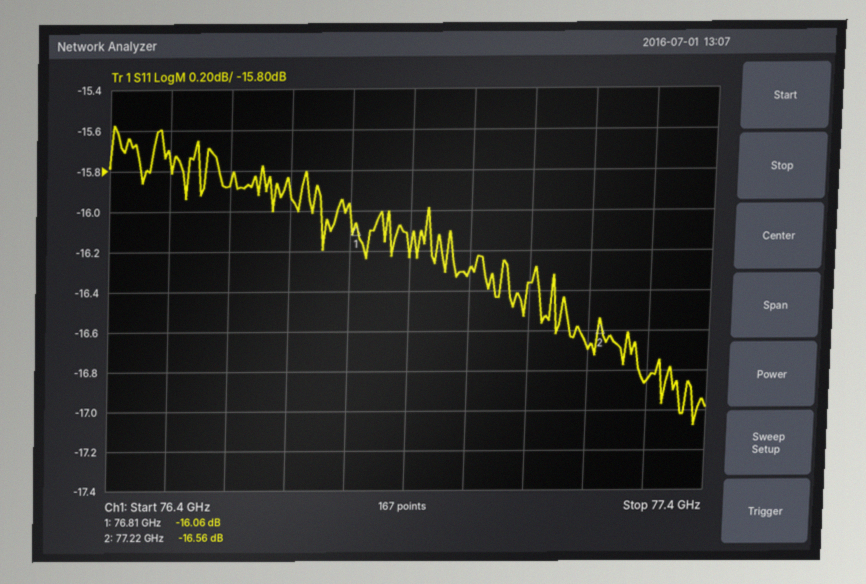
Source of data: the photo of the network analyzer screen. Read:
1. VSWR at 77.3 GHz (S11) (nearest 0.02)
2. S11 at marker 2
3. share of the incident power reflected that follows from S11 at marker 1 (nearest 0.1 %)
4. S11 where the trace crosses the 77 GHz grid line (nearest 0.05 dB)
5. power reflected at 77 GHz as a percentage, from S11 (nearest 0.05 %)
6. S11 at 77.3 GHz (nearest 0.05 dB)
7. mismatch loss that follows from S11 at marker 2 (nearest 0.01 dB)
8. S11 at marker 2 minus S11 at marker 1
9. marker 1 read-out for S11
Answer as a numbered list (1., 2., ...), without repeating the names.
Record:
1. 1.34
2. -16.56 dB
3. 2.5 %
4. -16.30 dB
5. 2.35 %
6. -16.85 dB
7. 0.10 dB
8. -0.50 dB
9. -16.06 dB
